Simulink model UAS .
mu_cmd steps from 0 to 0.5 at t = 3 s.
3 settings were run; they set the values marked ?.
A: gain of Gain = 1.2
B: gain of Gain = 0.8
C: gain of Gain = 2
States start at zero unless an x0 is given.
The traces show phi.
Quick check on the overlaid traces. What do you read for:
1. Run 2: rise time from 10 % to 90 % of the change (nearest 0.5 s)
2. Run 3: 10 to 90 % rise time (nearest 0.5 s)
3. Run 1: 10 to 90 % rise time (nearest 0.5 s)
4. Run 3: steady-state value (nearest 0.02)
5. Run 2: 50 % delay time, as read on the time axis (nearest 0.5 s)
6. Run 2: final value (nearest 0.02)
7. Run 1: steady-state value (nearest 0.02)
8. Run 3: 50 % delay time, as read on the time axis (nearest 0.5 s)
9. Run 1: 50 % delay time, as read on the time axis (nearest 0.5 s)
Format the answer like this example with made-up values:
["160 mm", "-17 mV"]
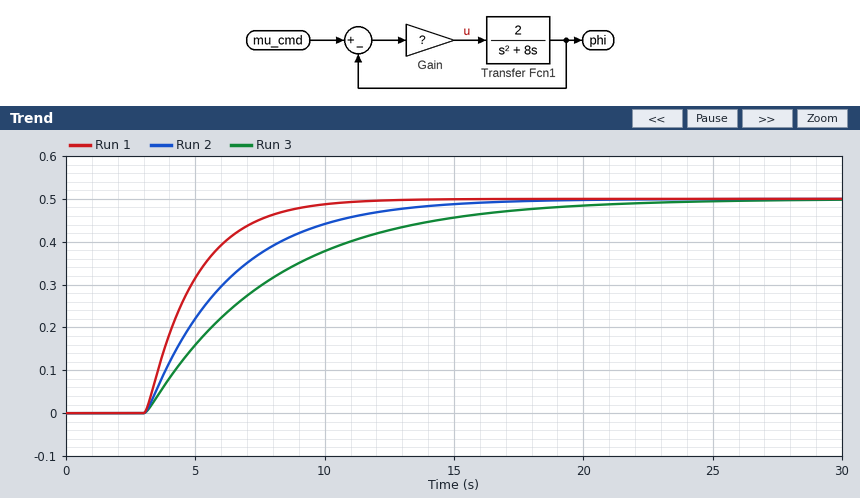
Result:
["7.0 s", "10.5 s", "4.0 s", "0.50", "5.5 s", "0.50", "0.50", "6.5 s", "4.5 s"]
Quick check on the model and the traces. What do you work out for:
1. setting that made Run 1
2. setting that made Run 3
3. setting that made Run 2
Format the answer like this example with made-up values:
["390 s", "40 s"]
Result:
["C", "B", "A"]
